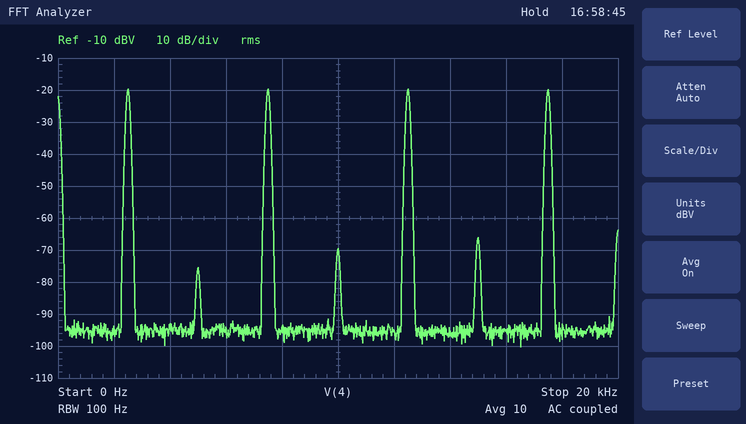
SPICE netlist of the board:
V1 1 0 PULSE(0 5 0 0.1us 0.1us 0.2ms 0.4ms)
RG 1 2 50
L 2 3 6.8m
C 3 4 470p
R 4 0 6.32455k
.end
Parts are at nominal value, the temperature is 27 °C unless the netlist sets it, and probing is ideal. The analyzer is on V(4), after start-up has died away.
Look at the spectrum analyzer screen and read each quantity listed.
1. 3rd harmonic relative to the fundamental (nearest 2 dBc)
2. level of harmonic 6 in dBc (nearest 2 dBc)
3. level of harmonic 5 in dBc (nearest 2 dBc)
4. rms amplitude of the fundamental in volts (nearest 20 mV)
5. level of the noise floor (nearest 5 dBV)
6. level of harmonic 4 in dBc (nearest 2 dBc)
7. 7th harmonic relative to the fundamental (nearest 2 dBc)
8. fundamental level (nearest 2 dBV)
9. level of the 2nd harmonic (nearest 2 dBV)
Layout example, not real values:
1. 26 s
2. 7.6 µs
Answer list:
1. 0 dBc
2. -46 dBc
3. 0 dBc
4. 100 mV
5. -95 dBV
6. -50 dBc
7. 0 dBc
8. -20 dBV
9. -76 dBV
